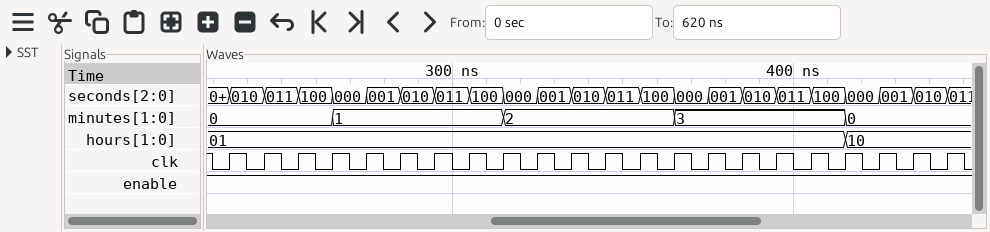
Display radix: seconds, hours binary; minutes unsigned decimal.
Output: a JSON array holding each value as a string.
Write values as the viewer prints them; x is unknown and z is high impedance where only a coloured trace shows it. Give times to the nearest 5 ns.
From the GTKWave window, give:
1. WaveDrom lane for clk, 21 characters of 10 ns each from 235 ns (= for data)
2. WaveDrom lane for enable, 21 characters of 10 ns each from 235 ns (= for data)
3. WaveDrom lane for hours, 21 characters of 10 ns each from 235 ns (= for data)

["{name: 'clk', wave: 'p....................'}", "{name: 'enable', wave: '1....................'}", "{name: 'hours', wave: '=.................=..', data: '01 10'}"]
